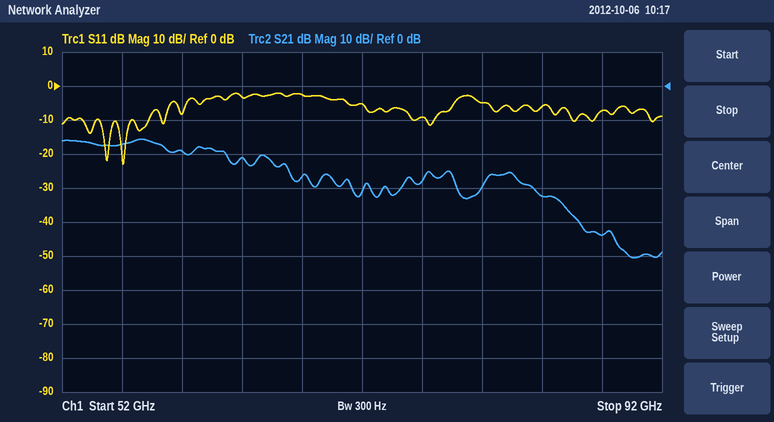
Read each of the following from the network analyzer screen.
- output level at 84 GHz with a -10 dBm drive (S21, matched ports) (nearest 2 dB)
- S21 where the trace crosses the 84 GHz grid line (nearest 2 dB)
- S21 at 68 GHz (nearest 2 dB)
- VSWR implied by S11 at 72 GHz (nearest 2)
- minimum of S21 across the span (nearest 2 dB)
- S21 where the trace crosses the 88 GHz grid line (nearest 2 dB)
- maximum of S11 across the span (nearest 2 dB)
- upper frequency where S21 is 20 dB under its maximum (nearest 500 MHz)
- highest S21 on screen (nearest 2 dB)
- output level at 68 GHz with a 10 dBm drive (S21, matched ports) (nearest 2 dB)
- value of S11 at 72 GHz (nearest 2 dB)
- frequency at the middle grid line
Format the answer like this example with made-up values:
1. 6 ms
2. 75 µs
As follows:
1. -42 dBm
2. -32 dB
3. -26 dB
4. 4
5. -50 dB
6. -44 dB
7. -2 dB
8. 85.5 GHz
9. -16 dB
10. -16 dBm
11. -6 dB
12. 72 GHz
